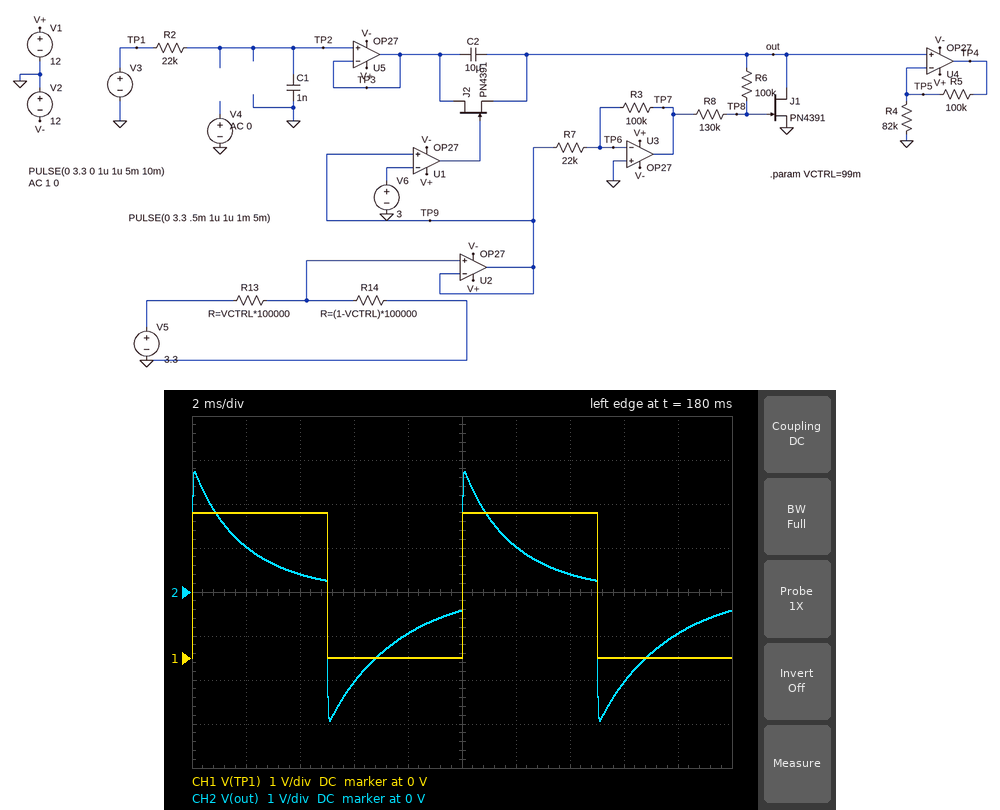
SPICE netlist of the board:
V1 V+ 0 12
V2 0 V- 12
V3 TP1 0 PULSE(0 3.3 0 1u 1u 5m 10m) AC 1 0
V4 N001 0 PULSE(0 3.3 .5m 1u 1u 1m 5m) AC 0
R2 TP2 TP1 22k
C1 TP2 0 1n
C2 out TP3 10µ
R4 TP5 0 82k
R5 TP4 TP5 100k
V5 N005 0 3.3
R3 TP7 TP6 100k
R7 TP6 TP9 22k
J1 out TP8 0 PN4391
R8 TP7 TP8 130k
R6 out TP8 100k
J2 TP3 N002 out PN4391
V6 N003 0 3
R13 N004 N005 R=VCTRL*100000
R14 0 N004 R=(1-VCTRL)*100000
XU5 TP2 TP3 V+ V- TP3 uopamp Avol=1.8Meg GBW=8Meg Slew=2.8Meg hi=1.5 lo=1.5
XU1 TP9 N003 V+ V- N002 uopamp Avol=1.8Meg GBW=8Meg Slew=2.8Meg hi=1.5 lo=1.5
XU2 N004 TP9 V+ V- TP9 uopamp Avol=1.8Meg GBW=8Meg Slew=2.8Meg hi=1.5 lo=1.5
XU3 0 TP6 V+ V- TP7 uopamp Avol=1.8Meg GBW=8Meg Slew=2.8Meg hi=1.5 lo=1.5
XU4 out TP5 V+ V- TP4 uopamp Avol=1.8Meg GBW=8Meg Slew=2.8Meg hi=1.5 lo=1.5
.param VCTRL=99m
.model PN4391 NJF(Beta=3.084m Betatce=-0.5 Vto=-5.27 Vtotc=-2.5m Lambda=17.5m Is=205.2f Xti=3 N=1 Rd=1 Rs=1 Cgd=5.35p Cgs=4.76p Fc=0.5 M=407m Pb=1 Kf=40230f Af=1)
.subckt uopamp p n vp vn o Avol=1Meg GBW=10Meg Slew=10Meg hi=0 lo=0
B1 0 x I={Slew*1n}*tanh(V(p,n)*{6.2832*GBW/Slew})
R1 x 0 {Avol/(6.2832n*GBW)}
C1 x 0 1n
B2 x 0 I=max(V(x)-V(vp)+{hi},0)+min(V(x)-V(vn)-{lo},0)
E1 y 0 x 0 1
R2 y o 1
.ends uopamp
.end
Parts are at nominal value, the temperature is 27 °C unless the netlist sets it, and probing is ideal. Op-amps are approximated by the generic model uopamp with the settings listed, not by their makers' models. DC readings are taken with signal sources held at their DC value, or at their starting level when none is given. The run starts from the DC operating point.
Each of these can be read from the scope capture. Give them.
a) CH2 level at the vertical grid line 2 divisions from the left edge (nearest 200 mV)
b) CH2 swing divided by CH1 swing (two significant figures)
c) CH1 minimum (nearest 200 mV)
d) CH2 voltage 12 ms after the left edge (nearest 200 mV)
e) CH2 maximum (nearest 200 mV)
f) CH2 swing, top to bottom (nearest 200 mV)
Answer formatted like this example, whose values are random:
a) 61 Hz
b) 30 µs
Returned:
a) 400 mV
b) 1.7
c) 0 V
d) 1.0 V
e) 2.8 V
f) 5.6 V
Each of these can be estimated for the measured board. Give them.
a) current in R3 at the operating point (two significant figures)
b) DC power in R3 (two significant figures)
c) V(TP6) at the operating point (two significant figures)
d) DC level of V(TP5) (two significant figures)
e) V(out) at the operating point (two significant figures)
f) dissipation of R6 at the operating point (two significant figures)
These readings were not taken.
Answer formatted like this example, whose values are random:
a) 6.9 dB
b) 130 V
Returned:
a) 110 µA
b) 1.2 mW
c) 540 mV
d) -11 mV
e) -11 mV
f) 210 µW
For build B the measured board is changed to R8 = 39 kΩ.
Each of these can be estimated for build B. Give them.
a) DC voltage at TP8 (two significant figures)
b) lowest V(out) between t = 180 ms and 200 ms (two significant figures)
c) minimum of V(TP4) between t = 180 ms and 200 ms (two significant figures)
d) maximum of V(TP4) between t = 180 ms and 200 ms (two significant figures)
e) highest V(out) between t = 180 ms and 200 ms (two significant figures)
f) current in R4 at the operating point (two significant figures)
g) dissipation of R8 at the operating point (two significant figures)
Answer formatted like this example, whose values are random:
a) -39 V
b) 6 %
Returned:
a) -8.5 V
b) -3.5 V
c) -7.7 V
d) -300 mV
e) -140 mV
f) 41 µA
g) 100 µW
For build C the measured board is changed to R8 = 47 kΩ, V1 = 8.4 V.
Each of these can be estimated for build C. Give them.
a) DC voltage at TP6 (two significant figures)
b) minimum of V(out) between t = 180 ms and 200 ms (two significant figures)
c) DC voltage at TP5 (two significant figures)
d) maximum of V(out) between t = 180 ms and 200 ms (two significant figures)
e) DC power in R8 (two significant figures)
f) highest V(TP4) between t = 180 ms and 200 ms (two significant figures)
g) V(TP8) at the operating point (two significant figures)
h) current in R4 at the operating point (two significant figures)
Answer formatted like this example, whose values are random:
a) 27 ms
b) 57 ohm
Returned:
a) 540 mV
b) -3.1 V
c) -2.9 V
d) 270 mV
e) 120 µW
f) 600 mV
g) -8.1 V
h) 36 µA
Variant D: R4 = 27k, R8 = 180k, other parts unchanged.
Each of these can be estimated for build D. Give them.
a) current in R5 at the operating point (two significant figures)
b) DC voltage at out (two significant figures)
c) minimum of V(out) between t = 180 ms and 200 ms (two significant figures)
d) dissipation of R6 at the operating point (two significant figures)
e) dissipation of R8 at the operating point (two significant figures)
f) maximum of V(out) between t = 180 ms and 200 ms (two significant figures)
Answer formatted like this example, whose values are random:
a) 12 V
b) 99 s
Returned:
a) 150 nA
b) -4.1 mV
c) -3.1 V
d) 140 µW
e) 250 µW
f) 3.0 V
